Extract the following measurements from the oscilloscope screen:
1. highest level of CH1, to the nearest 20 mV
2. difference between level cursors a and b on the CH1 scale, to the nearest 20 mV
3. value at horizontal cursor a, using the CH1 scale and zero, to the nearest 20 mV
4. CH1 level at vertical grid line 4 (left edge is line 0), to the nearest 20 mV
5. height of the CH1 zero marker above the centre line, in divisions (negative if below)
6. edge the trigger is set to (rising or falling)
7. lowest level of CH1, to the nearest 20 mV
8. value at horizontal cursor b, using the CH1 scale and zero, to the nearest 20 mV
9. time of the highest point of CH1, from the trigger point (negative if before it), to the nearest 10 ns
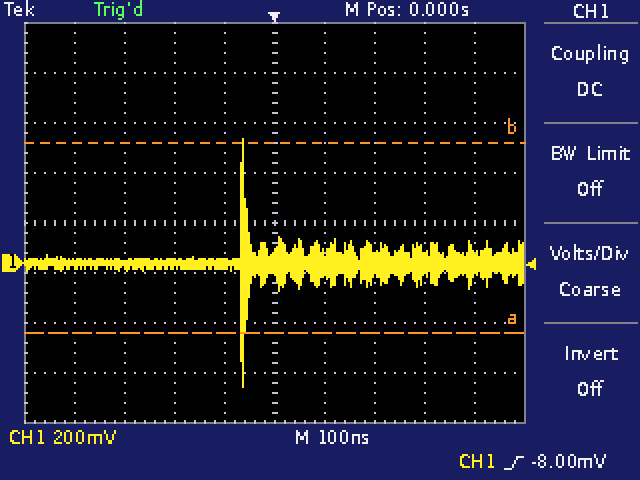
500 mV
760 mV
-280 mV
0 mV
-0.8 div
rising
-500 mV
480 mV
-60 ns
